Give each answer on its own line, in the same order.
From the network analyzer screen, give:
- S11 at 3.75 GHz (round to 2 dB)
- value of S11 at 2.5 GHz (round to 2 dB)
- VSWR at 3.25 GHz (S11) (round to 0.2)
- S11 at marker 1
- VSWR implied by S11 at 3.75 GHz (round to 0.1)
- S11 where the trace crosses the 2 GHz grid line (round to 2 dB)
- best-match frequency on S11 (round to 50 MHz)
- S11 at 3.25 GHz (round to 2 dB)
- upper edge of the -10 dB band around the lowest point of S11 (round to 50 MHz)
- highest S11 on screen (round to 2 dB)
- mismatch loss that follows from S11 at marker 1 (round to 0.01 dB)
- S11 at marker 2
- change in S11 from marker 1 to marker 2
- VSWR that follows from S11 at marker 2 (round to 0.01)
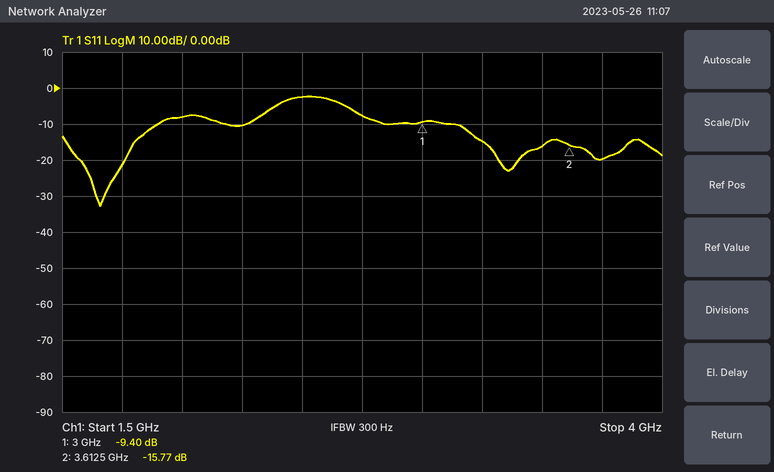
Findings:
-20 dB
-2 dB
1.4
-9.40 dB
1.2
-8 dB
1.65 GHz
-14 dB
1.90 GHz
-2 dB
0.53 dB
-15.77 dB
-6.37 dB
1.39
